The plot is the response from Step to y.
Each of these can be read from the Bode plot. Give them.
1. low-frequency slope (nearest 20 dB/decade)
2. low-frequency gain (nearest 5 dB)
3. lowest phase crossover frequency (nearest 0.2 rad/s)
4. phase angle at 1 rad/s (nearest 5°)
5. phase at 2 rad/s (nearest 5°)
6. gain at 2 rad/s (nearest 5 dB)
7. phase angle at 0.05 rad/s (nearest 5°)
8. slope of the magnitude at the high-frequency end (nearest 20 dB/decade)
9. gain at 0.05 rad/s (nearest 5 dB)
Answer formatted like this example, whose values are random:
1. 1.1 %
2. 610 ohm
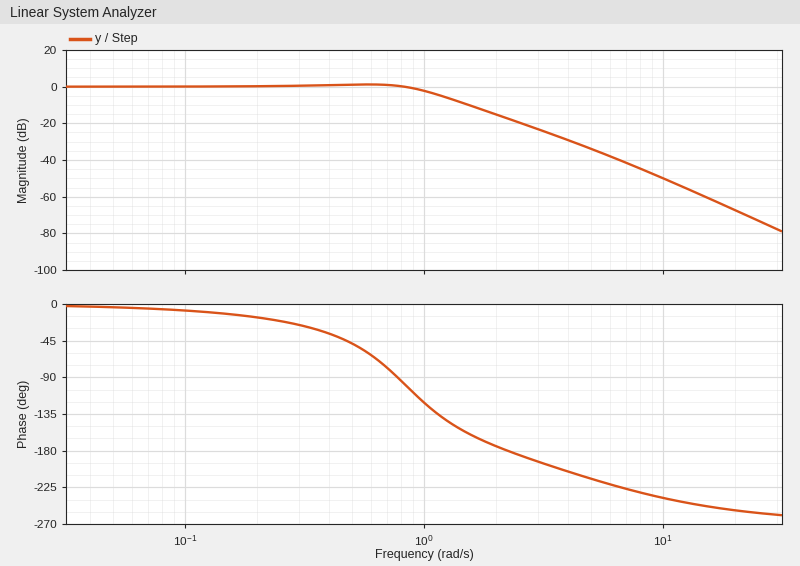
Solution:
1. 0 dB/decade
2. 0 dB
3. 2.2 rad/s
4. -120°
5. -175°
6. -15 dB
7. -5°
8. -60 dB/decade
9. 0 dB
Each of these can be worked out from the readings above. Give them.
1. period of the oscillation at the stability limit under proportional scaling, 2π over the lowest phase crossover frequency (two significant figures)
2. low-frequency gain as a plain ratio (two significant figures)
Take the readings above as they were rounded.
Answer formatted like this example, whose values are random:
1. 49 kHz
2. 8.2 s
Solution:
1. 2.9 s
2. 1.0
